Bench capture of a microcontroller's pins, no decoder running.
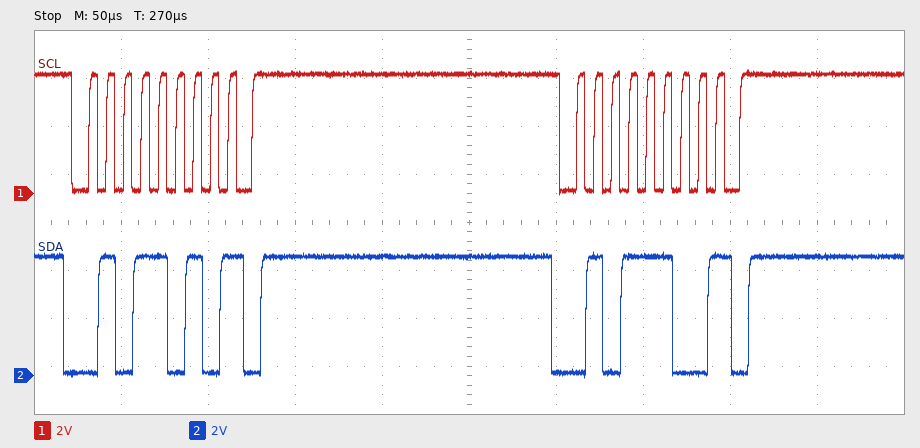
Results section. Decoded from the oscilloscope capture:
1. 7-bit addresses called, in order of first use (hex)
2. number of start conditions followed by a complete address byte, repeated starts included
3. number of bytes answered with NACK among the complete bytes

0x2D 0x2E
2
2
